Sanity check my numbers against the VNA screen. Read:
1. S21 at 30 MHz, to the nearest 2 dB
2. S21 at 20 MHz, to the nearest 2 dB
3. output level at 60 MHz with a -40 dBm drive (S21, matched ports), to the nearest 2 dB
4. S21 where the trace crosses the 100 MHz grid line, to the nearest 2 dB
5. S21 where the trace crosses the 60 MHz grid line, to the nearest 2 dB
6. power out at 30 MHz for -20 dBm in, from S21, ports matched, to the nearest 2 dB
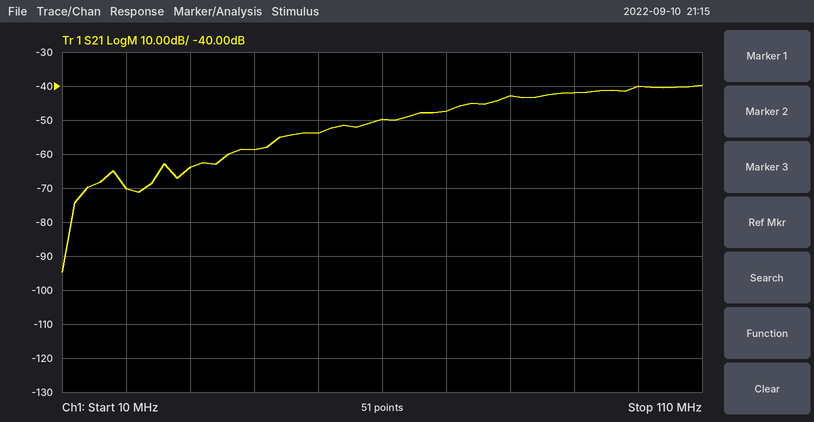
-64 dB
-70 dB
-90 dBm
-40 dB
-50 dB
-84 dBm
